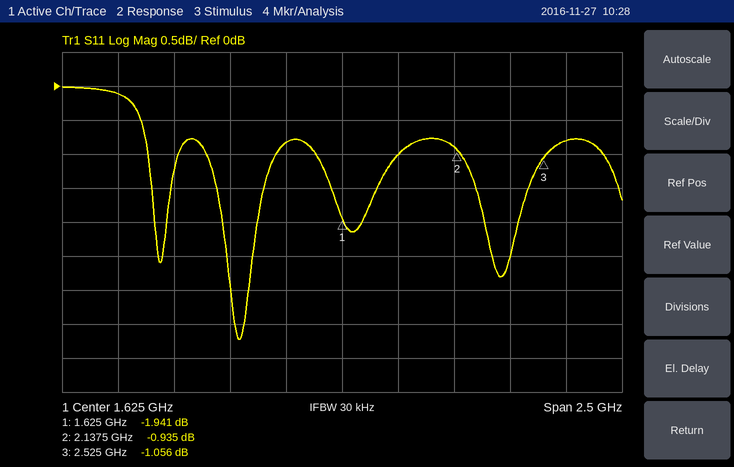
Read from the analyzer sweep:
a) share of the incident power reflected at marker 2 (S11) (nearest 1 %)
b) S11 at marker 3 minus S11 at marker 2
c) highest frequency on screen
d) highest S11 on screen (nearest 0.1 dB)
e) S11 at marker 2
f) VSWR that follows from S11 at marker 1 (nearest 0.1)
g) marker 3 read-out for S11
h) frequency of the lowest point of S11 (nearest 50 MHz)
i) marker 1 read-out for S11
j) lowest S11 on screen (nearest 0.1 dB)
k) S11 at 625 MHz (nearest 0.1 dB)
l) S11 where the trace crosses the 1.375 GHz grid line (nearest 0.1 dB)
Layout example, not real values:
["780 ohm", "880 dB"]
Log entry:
["81 %", "-0.121 dB", "2.875 GHz", "0.0 dB", "-0.935 dB", "9.0", "-1.056 dB", "1.15 GHz", "-1.941 dB", "-3.7 dB", "-0.1 dB", "-0.8 dB"]
